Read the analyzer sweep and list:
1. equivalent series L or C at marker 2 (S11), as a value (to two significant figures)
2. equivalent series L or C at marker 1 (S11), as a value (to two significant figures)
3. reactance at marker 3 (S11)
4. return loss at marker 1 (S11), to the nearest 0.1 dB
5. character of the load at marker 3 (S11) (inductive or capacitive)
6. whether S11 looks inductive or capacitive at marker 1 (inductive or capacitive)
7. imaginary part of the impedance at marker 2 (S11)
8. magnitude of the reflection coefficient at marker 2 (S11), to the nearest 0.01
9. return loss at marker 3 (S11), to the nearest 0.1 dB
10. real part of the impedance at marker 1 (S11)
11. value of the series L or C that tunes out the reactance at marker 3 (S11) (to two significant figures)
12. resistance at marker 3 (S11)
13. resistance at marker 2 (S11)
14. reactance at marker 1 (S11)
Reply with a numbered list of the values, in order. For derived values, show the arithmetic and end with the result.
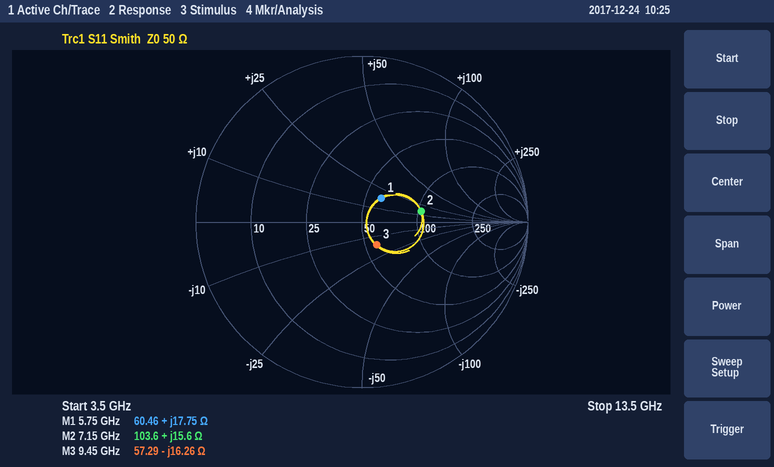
1. L = 15.6 Ω/(2π × 7.15 GHz) ≈ 347 pH, so 350 pH to two significant figures
2. L = 17.75 Ω/(2π × 5.75 GHz) ≈ 491 pH, so 490 pH to two significant figures
3. -16.26 Ω
4. 14.7 dB
5. capacitive
6. inductive
7. +15.6 Ω
8. 0.36
9. 15.7 dB
10. 60.46 Ω
11. L = 16.26 Ω/(2π × 9.45 GHz) ≈ 274 pH, so 270 pH to two significant figures
12. 57.29 Ω
13. 103.6 Ω
14. +17.75 Ω
